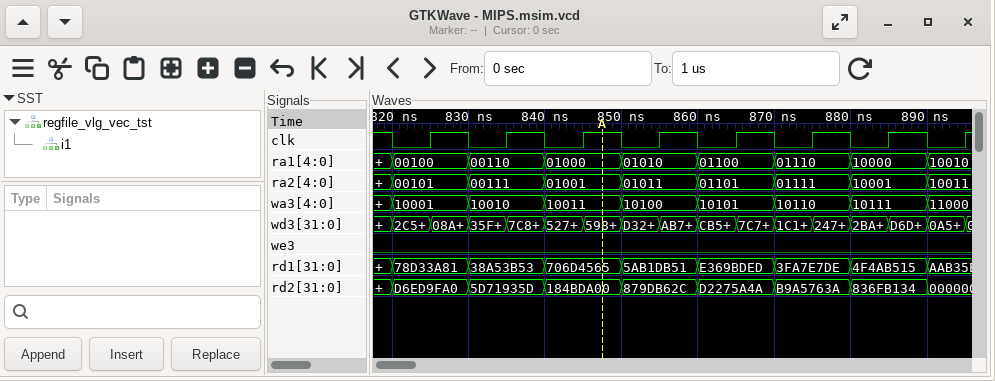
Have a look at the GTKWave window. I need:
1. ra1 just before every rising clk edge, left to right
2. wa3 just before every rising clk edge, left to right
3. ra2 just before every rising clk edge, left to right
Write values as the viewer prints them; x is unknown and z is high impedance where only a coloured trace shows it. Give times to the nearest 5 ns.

00100, 00110, 01000, 01010, 01100, 01110, 10000, 10010
10001, 10010, 10011, 10100, 10101, 10110, 10111, 11000
00101, 00111, 01001, 01011, 01101, 01111, 10001, 10011
